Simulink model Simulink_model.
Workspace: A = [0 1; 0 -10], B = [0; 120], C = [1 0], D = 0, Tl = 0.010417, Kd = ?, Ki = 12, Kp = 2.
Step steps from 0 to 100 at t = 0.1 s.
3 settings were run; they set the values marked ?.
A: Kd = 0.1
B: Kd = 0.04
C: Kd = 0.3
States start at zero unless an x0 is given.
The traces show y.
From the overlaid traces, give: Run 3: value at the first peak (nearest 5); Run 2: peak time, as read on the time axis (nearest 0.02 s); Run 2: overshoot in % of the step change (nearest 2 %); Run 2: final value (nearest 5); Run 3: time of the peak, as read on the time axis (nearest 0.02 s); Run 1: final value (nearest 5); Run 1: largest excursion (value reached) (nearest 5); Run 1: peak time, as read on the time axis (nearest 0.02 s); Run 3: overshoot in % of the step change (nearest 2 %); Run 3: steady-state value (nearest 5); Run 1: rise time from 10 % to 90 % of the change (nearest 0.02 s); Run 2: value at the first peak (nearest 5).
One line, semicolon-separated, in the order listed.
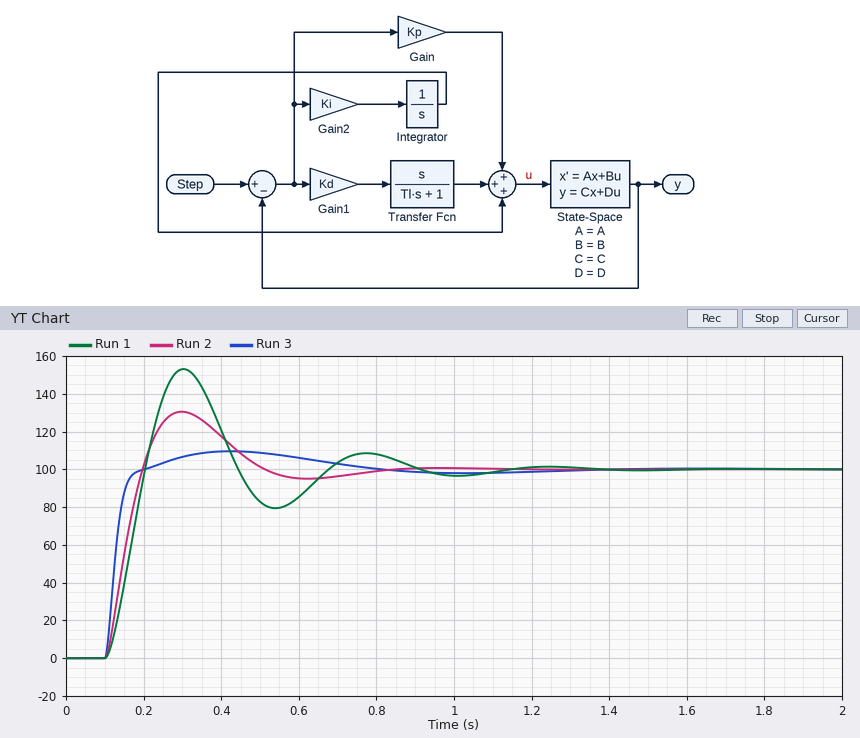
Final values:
110; 0.30 s; 30 %; 100; 0.42 s; 100; 155; 0.30 s; 10 %; 100; 0.08 s; 130
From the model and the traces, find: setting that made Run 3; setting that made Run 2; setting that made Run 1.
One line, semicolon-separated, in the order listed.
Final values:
C; A; B
